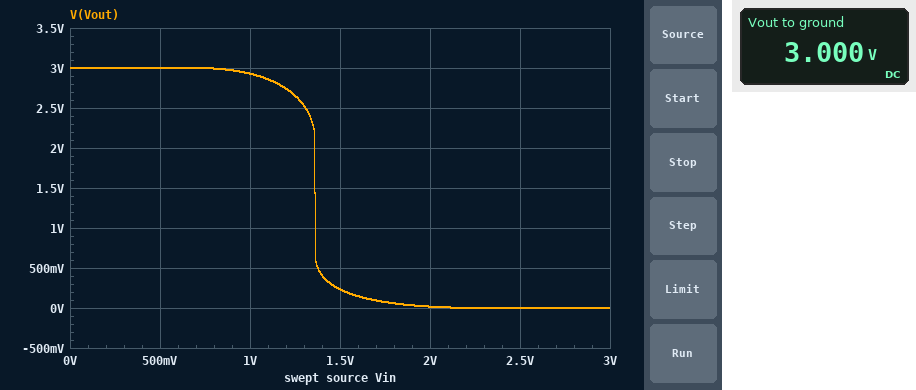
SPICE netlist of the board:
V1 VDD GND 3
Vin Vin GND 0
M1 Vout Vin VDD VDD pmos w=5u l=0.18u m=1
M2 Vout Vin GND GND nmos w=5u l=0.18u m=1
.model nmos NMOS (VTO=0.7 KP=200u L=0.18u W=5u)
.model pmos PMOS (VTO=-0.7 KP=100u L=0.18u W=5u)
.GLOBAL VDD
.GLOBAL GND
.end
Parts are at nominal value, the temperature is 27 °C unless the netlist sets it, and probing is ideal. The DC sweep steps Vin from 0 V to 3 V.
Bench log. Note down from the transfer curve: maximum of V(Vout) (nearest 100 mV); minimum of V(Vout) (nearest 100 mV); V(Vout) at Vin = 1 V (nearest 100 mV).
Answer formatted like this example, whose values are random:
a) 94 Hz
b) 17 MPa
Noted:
a) 3.0 V
b) 0 V
c) 2.9 V
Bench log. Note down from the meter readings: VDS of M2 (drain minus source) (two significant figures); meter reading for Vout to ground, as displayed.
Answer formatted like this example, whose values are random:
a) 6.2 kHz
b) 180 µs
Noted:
a) 3.0 V
b) 3.000 V
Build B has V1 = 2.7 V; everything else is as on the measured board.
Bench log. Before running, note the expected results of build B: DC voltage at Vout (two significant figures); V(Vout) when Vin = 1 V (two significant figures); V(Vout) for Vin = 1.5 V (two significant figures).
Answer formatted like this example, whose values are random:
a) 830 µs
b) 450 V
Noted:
a) 2.7 V
b) 2.6 V
c) 82 mV
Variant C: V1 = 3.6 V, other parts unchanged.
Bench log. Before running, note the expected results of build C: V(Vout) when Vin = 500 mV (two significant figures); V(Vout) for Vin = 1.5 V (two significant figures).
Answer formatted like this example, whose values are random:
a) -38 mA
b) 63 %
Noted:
a) 3.6 V
b) 3.0 V
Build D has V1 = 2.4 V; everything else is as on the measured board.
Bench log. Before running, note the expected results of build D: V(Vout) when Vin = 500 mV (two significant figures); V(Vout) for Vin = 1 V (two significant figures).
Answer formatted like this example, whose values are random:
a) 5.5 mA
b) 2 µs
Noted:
a) 2.4 V
b) 2.3 V
